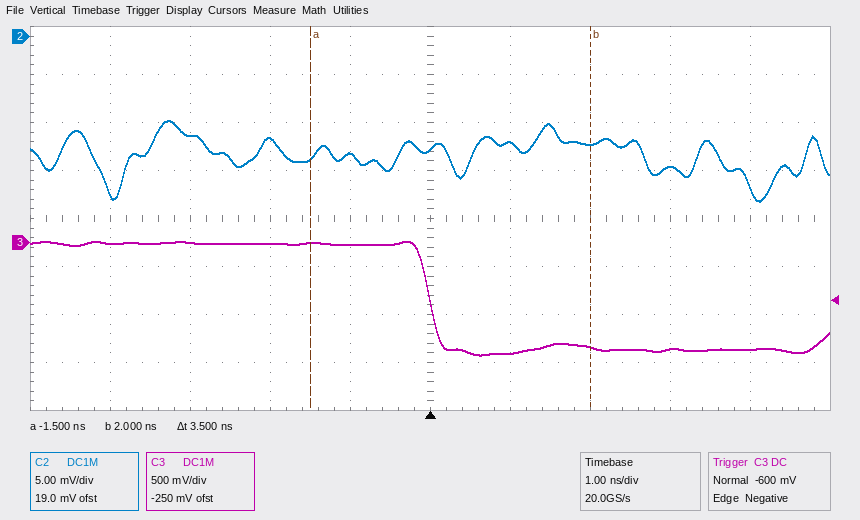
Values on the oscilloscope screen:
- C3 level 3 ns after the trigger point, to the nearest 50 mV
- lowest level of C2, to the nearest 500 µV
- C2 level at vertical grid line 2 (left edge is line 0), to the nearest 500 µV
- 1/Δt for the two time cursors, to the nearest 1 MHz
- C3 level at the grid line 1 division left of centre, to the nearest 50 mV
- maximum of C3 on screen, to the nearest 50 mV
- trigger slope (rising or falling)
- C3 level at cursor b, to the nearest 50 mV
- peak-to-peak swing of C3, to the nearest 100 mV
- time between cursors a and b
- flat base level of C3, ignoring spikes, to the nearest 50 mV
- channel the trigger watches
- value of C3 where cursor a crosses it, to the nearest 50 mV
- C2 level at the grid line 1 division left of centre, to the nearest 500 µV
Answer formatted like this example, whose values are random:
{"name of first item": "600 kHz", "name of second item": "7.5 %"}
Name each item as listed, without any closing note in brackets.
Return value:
{"C3 level 3 ns after the trigger point, to the nearest 50 mV": "-1.10 V", "lowest level of C2, to the nearest 500 µV": "-17.0 mV", "C2 level at vertical grid line 2 (left edge is line 0), to the nearest 500 µV": "-10.5 mV", "1/Δt for the two time cursors, to the nearest 1 MHz": "286 MHz", "C3 level at the grid line 1 division left of centre, to the nearest 50 mV": "0 mV", "maximum of C3 on screen, to the nearest 50 mV": "0 mV", "trigger slope": "falling", "C3 level at cursor b, to the nearest 50 mV": "-1.10 V", "peak-to-peak swing of C3, to the nearest 100 mV": "1.20 V", "time between cursors a and b": "3.5 ns", "flat base level of C3, ignoring spikes, to the nearest 50 mV": "-1.10 V", "channel the trigger watches": "C3", "value of C3 where cursor a crosses it, to the nearest 50 mV": "0 mV", "C2 level at the grid line 1 division left of centre, to the nearest 500 µV": "-12.5 mV"}
